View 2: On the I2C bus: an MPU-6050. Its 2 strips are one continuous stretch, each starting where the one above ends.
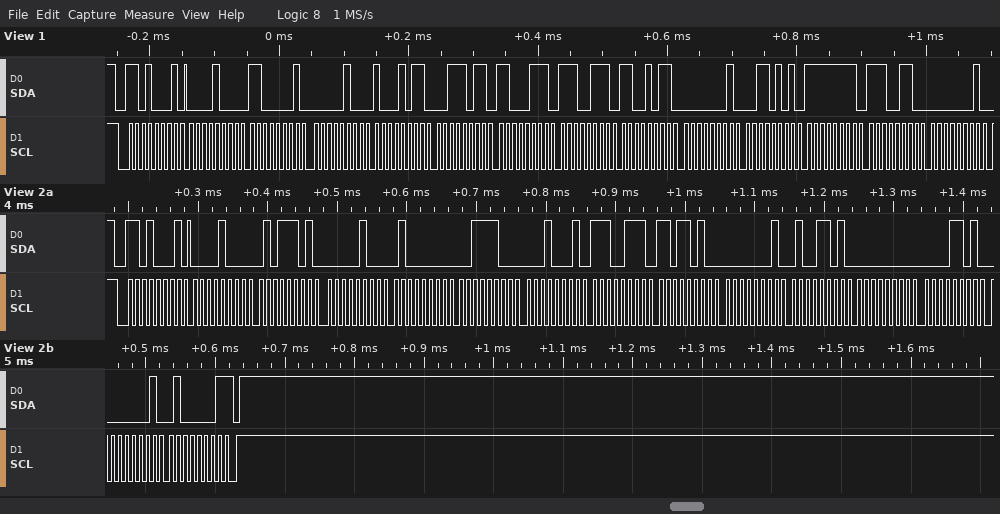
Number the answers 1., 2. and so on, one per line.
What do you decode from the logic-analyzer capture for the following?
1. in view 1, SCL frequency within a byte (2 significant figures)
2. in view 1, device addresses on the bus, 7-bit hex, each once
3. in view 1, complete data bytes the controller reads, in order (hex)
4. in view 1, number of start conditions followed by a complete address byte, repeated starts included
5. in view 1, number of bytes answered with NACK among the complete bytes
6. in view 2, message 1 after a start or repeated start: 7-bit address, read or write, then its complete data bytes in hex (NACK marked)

1. 100 kHz
2. 0x68
3. 08 C1 04 8B 3B C7 E7 CB 01 35 FF E6 01
4. 1
5. 0
6. 0x68 read: 08 5D 04 40 3C 11 E7 DA 01 4D 00 0D 01 41 NACK
